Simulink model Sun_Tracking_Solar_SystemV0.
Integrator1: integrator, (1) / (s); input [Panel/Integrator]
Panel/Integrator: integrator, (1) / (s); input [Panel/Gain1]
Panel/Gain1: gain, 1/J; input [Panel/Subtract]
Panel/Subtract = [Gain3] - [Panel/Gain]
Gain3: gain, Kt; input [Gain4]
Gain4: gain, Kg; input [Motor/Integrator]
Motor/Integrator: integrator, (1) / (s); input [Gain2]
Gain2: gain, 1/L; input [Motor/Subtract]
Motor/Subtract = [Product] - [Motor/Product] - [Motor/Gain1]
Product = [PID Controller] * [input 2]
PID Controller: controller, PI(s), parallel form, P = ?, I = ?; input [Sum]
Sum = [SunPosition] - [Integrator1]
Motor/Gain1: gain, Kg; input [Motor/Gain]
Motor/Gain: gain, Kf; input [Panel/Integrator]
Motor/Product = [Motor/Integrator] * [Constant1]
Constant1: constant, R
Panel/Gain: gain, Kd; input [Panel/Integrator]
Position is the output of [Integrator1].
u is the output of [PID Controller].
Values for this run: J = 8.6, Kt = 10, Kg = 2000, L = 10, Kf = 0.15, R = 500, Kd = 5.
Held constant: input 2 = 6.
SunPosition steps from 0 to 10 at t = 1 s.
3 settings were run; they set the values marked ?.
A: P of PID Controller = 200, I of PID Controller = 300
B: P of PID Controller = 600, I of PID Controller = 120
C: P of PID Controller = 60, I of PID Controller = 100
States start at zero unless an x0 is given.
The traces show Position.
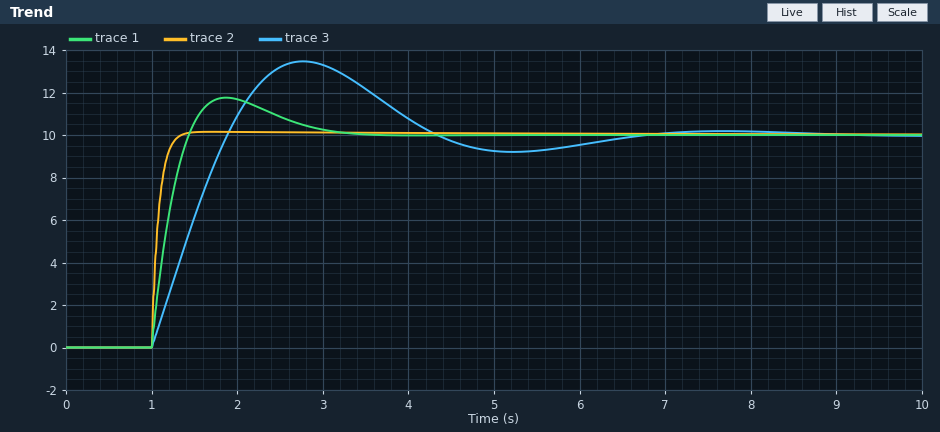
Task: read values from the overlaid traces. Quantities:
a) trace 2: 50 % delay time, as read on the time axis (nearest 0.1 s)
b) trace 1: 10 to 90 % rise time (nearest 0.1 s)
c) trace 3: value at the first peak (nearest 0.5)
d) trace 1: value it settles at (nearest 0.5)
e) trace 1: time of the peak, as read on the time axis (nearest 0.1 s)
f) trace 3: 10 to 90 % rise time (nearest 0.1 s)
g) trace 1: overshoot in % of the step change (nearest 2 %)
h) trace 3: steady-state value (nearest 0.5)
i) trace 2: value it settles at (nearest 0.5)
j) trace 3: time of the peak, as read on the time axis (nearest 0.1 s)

1.1 s
0.3 s
13.5
10.0
1.9 s
0.7 s
18 %
10.0
10.0
2.8 s
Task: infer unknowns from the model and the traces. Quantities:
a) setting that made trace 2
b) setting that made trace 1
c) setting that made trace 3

B
A
C
